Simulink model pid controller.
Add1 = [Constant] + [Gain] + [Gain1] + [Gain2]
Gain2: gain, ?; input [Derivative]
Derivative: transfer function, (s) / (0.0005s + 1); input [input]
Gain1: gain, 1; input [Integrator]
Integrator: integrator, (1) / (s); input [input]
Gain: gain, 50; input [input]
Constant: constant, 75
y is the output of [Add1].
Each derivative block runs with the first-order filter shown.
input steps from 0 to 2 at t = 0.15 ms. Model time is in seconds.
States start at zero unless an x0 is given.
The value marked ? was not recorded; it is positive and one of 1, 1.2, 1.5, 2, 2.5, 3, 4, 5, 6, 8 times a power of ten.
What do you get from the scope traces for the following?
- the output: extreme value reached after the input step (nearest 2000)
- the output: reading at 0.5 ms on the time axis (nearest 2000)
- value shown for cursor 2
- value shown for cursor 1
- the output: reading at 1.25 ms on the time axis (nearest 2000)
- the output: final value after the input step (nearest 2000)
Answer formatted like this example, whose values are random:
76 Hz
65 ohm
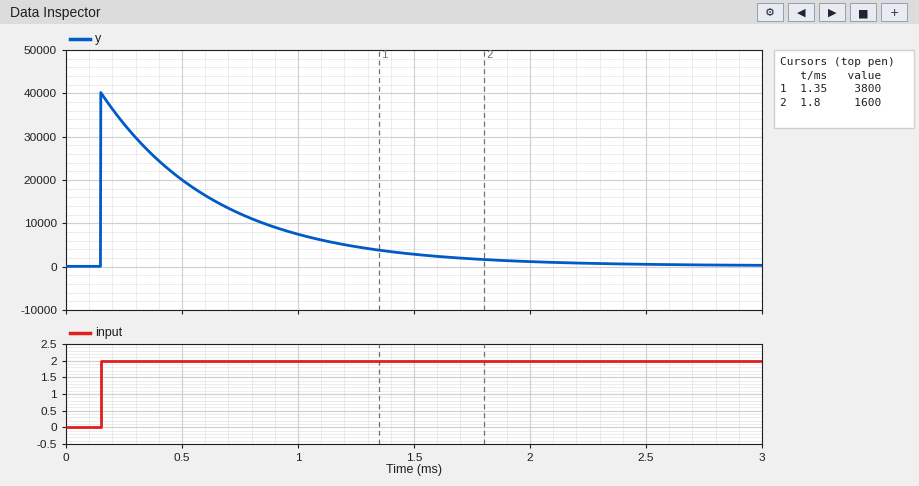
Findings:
40000
20000
1600
3800
4000
0
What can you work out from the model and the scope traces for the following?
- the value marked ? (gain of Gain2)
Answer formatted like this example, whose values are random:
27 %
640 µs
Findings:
10
